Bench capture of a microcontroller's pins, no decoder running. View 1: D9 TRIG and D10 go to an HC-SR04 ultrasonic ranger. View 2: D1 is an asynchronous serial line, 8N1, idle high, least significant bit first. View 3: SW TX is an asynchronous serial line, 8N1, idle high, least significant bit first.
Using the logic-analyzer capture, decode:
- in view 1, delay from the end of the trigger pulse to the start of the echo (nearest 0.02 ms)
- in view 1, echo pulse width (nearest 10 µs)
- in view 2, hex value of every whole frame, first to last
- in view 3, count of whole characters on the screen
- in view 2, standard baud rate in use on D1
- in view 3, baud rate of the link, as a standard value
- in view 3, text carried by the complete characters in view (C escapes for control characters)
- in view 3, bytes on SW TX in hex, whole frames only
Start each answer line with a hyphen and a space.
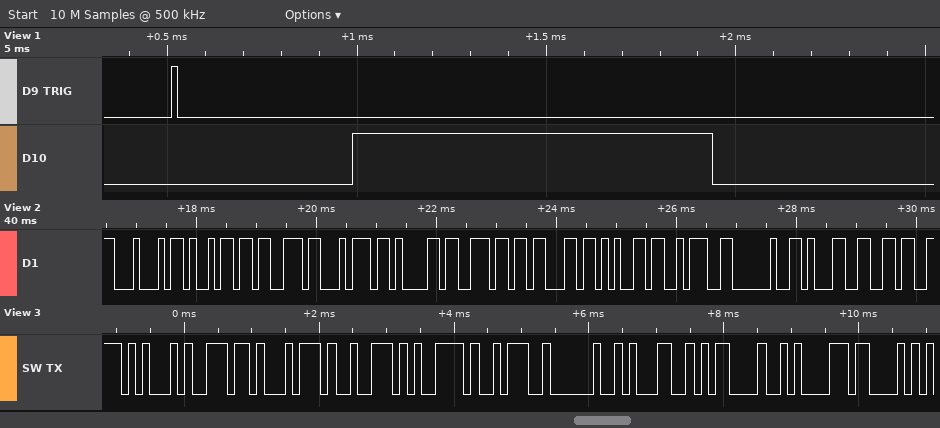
- 0.46 ms
- 950 µs
- 44 69 73 74 61 6E 63 65 3A 20 31 36
- 11
- 9600 baud
- 9600 baud
- "Entry: 1\r\nC"
- 45 6E 74 72 79 3A 20 31 0D 0A 43
